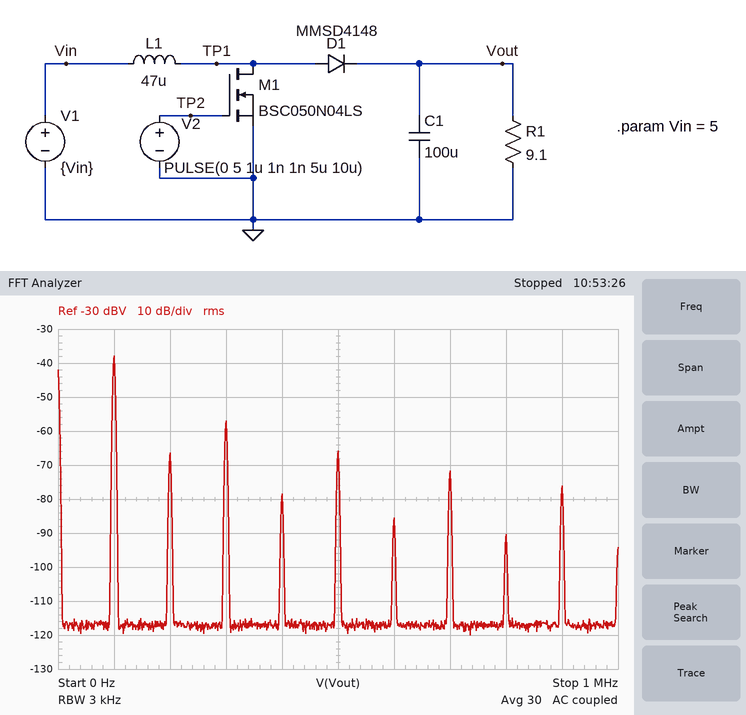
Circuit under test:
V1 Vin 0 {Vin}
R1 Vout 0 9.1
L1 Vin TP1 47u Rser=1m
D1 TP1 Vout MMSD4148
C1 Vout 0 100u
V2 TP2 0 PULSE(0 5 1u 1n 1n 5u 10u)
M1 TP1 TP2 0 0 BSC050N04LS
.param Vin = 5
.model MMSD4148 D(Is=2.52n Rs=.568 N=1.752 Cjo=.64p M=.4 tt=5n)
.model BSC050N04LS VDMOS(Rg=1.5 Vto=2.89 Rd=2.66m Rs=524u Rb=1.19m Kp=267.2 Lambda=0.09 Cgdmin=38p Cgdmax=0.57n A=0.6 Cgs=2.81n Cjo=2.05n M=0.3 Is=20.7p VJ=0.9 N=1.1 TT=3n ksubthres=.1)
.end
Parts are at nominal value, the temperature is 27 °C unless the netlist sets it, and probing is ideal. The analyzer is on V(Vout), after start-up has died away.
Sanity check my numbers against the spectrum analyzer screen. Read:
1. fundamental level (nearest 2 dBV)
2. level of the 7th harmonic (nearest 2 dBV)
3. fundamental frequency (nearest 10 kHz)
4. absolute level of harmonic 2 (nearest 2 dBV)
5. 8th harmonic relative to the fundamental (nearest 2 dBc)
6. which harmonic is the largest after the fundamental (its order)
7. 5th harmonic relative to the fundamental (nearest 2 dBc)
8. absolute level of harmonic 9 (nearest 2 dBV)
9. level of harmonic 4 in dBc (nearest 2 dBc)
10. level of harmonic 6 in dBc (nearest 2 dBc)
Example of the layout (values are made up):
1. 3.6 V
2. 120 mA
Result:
1. -38 dBV
2. -72 dBV
3. 100 kHz
4. -66 dBV
5. -52 dBc
6. 3
7. -28 dBc
8. -76 dBV
9. -40 dBc
10. -48 dBc
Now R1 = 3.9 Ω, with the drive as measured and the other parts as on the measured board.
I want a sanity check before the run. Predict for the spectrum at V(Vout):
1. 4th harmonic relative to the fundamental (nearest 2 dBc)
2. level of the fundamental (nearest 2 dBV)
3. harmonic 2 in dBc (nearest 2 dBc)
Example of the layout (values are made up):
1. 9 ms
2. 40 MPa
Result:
1. -46 dBc
2. -32 dBV
3. -34 dBc
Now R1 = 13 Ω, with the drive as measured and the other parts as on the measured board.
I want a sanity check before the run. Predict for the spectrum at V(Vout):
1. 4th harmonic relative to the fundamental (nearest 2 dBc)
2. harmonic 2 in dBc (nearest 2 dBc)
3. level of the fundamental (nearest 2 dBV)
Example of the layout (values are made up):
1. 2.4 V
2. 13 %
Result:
1. -38 dBc
2. -26 dBc
3. -40 dBV
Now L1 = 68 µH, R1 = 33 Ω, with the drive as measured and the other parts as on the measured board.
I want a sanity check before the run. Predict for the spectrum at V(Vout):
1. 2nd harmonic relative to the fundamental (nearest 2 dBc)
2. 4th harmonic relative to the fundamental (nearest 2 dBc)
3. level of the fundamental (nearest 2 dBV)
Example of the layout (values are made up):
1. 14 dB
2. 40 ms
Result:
1. -22 dBc
2. -34 dBc
3. -48 dBV
